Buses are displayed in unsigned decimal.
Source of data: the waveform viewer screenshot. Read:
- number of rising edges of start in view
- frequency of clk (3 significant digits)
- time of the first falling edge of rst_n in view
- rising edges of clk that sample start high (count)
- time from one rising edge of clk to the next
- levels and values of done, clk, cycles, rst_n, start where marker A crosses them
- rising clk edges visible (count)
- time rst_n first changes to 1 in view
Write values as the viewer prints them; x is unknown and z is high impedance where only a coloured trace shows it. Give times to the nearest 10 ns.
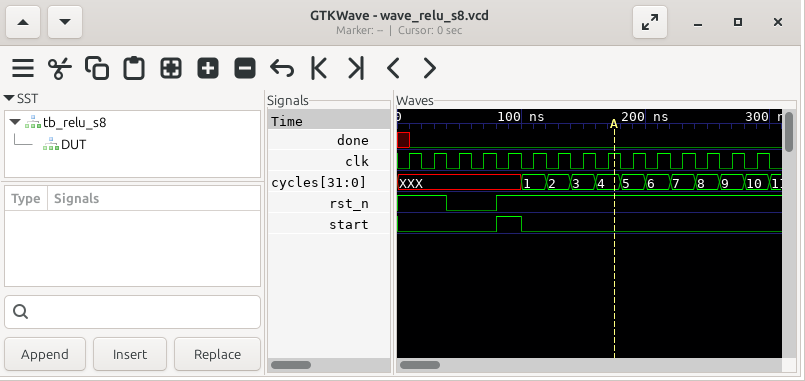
1
50.0 MHz
40 ns
1
20 ns
done=0, clk=1, cycles=4, rst_n=1, start=0
15
80 ns
